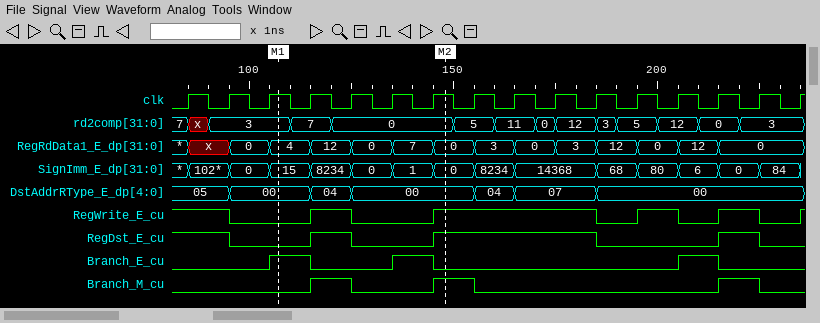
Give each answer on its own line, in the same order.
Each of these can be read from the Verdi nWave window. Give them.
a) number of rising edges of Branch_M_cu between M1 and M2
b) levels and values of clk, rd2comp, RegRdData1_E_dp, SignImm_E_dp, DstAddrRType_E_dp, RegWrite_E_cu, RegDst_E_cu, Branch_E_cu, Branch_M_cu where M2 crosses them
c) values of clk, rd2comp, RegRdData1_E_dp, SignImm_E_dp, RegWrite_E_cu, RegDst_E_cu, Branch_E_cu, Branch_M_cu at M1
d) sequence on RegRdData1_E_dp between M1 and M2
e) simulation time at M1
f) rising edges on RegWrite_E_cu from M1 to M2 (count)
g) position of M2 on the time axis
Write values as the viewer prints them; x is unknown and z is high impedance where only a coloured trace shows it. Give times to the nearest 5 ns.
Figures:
2
clk=1, rd2comp=0, RegRdData1_E_dp=0, SignImm_E_dp=0, DstAddrRType_E_dp=00, RegWrite_E_cu=1, RegDst_E_cu=1, Branch_E_cu=0, Branch_M_cu=1
clk=1, rd2comp=3, RegRdData1_E_dp=4, SignImm_E_dp=15, RegWrite_E_cu=0, RegDst_E_cu=0, Branch_E_cu=1, Branch_M_cu=0
4, 12, 0, 7, 0
105 ns
2
150 ns
